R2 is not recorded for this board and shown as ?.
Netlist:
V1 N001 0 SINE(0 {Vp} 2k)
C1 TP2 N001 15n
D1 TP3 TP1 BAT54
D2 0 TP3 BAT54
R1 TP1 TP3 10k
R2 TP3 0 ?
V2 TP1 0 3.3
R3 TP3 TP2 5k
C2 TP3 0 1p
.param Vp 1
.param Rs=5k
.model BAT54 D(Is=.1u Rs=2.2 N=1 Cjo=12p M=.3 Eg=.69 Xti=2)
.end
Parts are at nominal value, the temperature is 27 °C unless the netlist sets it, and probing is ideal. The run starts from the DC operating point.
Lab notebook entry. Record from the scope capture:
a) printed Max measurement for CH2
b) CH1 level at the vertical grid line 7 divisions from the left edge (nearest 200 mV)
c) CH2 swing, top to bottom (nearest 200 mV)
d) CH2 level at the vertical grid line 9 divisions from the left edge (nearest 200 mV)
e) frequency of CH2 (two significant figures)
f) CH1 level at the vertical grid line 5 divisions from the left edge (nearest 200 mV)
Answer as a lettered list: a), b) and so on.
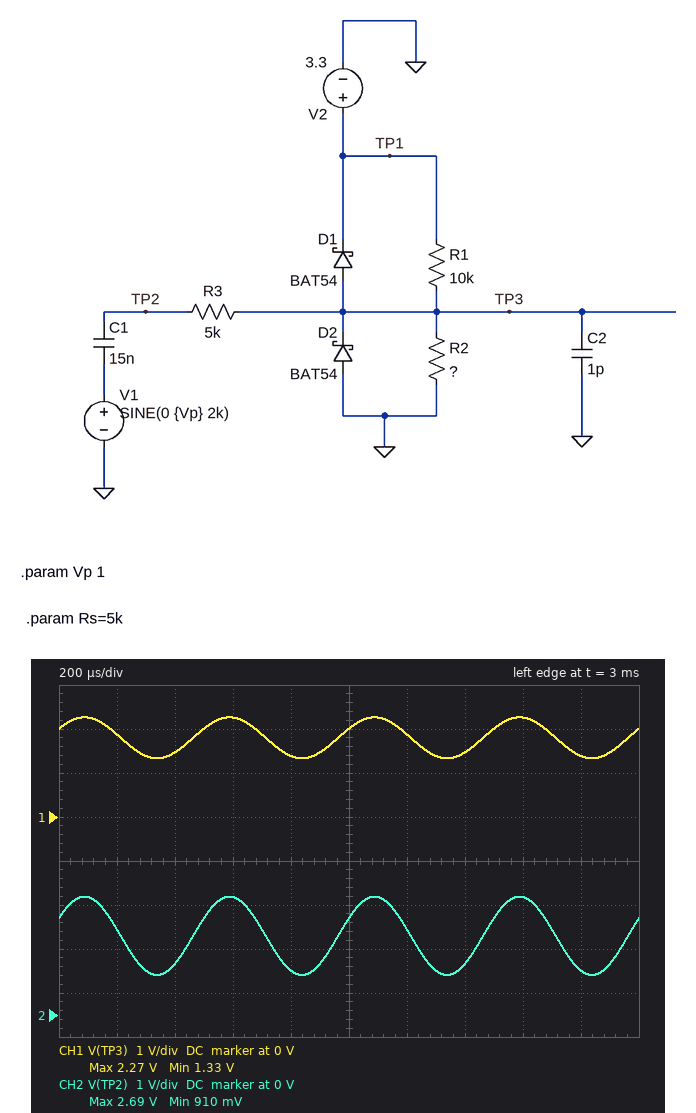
a) 2.69 V
b) 1.4 V
c) 1.8 V
d) 1.0 V
e) 2.0 kHz
f) 2.0 V
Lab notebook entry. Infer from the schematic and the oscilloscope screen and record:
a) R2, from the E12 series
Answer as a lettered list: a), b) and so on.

a) 12 kΩ
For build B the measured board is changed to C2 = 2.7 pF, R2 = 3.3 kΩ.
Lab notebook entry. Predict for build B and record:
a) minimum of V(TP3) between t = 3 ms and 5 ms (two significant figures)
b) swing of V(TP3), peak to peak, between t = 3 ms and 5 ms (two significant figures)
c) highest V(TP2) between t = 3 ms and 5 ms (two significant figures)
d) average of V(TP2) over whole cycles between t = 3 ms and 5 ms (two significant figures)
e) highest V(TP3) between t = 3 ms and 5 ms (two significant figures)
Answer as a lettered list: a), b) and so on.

a) 550 mV
b) 540 mV
c) 1.6 V
d) 820 mV
e) 1.1 V
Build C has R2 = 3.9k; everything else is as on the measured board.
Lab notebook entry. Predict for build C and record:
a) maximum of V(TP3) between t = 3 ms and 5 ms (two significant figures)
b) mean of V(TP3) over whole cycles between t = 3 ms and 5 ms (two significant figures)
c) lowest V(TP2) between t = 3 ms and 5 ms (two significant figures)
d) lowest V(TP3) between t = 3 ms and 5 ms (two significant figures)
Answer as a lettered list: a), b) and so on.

a) 1.2 V
b) 930 mV
c) 99 mV
d) 630 mV
